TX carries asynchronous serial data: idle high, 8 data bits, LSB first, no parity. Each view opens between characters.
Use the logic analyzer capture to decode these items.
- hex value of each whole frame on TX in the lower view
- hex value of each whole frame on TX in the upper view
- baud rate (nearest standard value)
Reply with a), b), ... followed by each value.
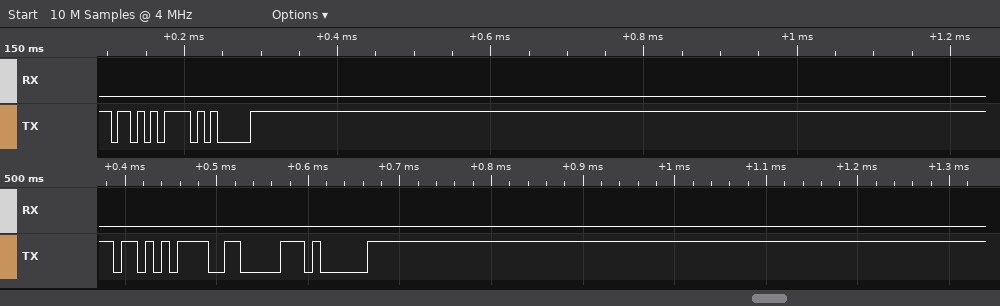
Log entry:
a) AB, 06, 81
b) AB, 05
c) 115200 baud
